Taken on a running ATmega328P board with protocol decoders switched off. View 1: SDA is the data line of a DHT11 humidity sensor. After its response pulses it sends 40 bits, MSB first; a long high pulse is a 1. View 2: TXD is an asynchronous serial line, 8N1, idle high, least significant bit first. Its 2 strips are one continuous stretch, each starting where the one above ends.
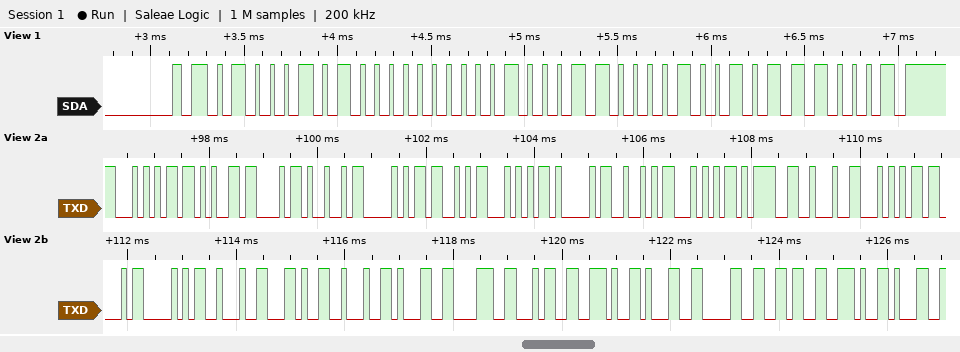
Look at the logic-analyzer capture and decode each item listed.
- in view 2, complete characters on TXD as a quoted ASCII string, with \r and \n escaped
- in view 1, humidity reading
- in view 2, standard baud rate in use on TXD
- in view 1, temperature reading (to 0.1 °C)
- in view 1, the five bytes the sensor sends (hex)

"T+CIPSTART=\"TCP\",\"184.106.1"
69 %
9600 baud
35.9 °C
45 00 23 09 71
